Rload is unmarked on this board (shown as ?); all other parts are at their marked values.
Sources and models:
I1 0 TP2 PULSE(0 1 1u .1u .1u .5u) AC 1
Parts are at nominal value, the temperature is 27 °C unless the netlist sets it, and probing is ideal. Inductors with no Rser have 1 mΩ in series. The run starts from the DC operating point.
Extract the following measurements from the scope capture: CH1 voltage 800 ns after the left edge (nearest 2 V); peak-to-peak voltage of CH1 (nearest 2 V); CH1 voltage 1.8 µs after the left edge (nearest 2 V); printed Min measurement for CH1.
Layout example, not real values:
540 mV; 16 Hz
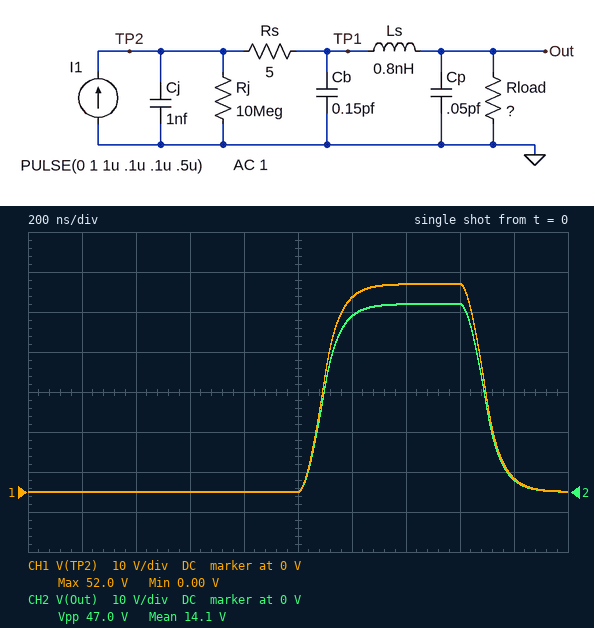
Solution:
0 V; 52 V; 4 V; 0.00 V
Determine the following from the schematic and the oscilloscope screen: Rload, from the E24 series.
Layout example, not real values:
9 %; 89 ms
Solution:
47 Ω
